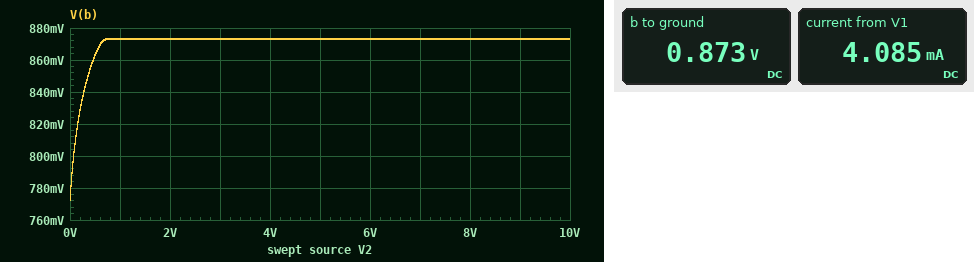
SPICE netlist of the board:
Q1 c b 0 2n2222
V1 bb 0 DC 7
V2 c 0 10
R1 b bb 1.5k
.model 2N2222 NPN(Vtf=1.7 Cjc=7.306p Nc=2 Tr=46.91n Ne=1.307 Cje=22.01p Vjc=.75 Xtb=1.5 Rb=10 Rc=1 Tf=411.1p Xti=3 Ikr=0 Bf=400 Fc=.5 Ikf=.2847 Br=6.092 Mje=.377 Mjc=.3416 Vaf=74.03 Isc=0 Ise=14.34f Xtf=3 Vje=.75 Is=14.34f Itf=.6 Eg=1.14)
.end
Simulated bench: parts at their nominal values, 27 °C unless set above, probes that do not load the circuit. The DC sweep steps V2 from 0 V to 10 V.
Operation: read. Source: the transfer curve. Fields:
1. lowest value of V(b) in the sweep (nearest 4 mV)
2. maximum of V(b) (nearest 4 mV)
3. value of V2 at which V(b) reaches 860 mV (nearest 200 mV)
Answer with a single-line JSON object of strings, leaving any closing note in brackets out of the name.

{"lowest value of V(b) in the sweep": "772 mV", "maximum of V(b)": "872 mV", "value of V2 at which V(b) reaches 860 mV": "400 mV"}
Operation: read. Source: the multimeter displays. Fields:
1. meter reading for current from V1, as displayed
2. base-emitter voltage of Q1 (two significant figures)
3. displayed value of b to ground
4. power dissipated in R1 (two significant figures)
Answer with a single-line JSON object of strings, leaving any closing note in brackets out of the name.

{"meter reading for current from V1, as displayed": "4.085 mA", "base-emitter voltage of Q1": "870 mV", "displayed value of b to ground": "0.873 V", "power dissipated in R1": "25 mW"}
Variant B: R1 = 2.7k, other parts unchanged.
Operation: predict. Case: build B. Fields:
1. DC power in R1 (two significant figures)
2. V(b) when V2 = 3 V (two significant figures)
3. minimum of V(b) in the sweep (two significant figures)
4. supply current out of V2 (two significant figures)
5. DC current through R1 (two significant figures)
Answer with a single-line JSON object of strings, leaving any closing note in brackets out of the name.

{"DC power in R1": "14 mW", "V(b) when V2 = 3 V": "840 mV", "minimum of V(b) in the sweep": "740 mV", "supply current out of V2": "380 mA", "DC current through R1": "2.3 mA"}
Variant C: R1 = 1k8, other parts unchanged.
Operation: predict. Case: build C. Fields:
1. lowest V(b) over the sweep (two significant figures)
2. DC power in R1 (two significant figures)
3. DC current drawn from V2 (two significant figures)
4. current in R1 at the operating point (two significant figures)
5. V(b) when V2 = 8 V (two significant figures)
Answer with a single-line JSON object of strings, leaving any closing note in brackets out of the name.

{"lowest V(b) over the sweep": "760 mV", "DC power in R1": "21 mW", "DC current drawn from V2": "490 mA", "current in R1 at the operating point": "3.4 mA", "V(b) when V2 = 8 V": "860 mV"}
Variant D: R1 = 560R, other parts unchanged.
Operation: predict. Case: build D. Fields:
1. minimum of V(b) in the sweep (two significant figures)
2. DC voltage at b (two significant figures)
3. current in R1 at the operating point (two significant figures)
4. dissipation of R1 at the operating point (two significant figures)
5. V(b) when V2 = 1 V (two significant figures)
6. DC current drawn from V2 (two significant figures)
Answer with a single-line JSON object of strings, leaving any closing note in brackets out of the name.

{"minimum of V(b) in the sweep": "870 mV", "DC voltage at b": "970 mV", "current in R1 at the operating point": "11 mA", "dissipation of R1 at the operating point": "65 mW", "V(b) when V2 = 1 V": "960 mV", "DC current drawn from V2": "990 mA"}
